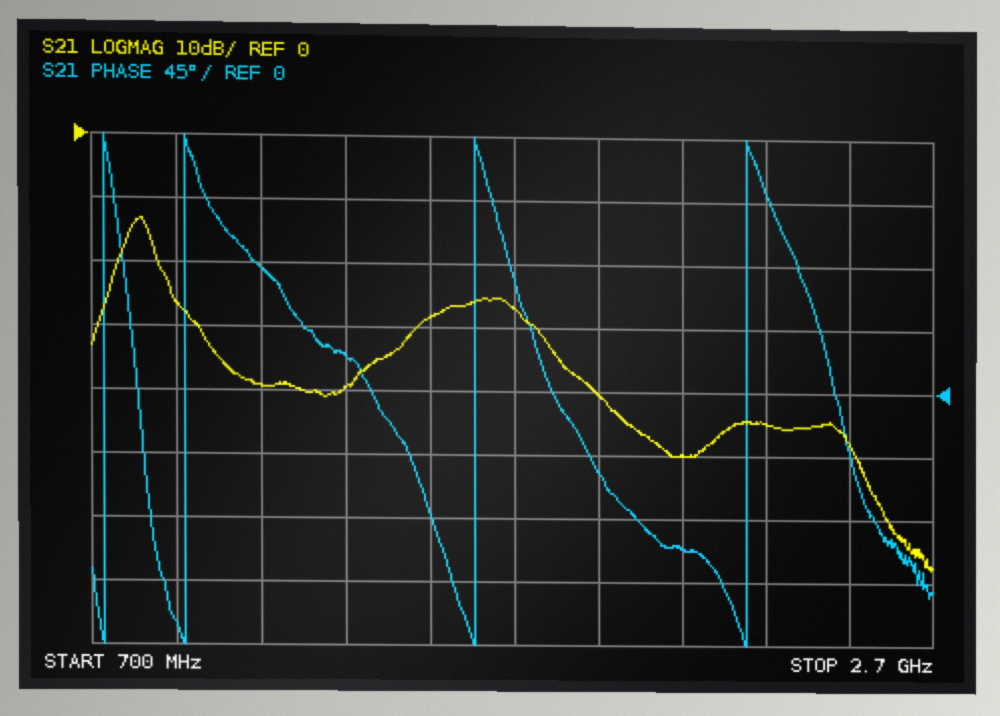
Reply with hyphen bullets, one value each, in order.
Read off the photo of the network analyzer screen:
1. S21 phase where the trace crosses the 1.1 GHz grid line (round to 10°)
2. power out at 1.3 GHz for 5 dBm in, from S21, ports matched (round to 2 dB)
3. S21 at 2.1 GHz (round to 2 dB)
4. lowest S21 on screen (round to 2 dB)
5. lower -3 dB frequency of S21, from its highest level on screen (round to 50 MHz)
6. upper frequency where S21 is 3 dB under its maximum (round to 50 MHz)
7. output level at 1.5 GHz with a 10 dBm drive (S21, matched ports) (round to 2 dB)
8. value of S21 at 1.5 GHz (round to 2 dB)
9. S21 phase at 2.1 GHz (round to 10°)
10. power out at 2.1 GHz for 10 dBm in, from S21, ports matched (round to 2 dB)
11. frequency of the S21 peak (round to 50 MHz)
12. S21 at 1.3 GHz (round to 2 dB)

- 90°
- -34 dBm
- -50 dB
- -68 dB
- 800 MHz
- 850 MHz
- -18 dBm
- -28 dB
- -110°
- -40 dBm
- 800 MHz
- -40 dB
